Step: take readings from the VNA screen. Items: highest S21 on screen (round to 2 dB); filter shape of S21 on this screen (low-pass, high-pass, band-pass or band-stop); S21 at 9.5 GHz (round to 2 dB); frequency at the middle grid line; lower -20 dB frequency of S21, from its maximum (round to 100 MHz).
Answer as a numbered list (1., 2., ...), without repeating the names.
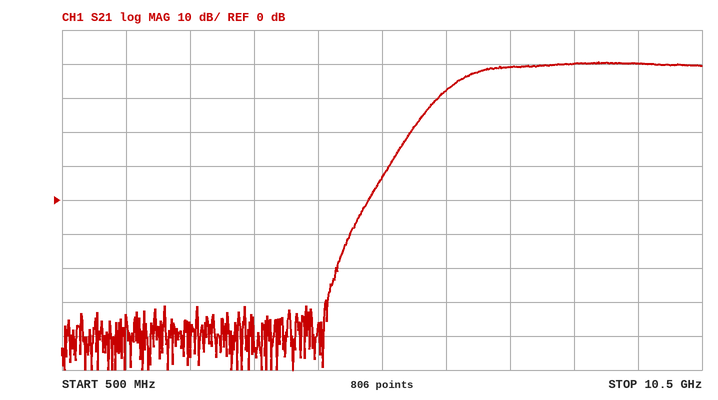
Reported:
1. 40 dB
2. high-pass
3. 40 dB
4. 5.5 GHz
5. 6.0 GHz
